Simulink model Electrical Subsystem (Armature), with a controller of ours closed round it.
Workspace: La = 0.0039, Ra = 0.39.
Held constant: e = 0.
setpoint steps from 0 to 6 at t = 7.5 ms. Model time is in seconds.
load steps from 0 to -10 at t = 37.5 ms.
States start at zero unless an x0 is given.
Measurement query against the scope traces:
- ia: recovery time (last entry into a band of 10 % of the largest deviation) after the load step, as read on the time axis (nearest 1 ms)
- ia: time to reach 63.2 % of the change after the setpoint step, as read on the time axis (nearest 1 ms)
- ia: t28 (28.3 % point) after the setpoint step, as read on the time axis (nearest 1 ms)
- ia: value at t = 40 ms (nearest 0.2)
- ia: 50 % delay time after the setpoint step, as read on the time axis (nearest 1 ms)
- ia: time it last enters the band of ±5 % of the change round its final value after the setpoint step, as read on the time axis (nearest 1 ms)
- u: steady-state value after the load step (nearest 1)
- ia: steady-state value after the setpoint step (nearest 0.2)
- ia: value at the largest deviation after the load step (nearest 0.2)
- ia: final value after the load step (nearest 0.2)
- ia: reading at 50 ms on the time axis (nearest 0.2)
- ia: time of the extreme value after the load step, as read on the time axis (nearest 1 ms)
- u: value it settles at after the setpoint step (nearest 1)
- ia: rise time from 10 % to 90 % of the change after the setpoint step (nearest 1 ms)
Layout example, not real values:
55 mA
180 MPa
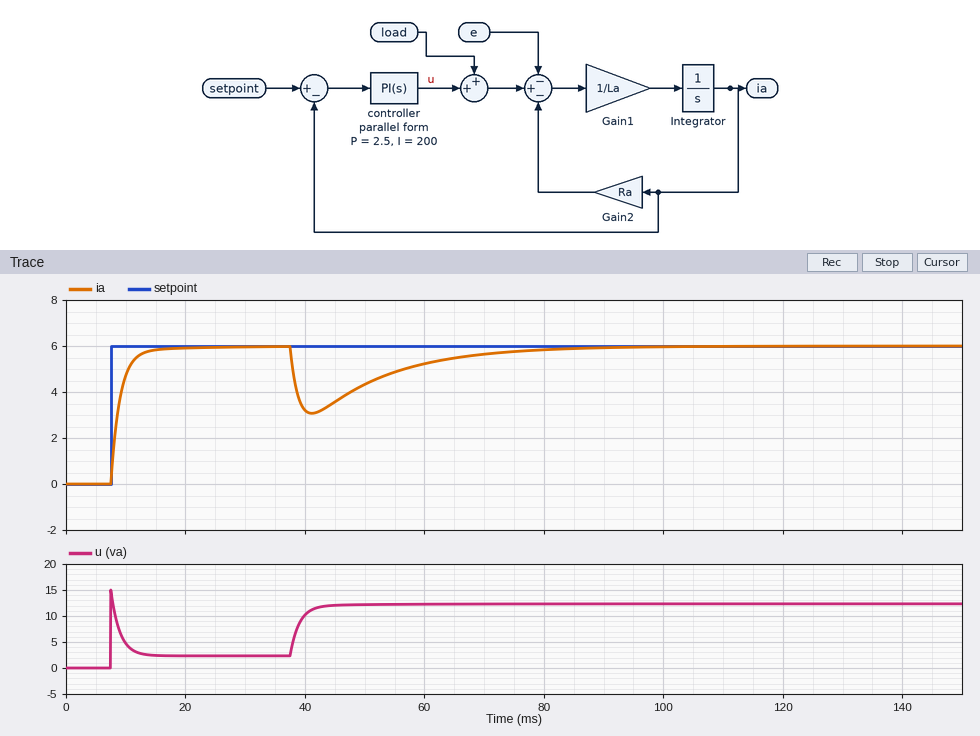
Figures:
73 ms
9 ms
8 ms
3.2
9 ms
13 ms
12
6.0
3.0
6.0
4.4
41 ms
2
4 ms
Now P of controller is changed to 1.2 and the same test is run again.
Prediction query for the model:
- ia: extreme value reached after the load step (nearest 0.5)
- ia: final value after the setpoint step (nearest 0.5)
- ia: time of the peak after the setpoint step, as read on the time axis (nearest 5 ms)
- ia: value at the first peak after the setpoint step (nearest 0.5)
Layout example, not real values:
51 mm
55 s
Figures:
1.5
6.0
20 ms
6.5
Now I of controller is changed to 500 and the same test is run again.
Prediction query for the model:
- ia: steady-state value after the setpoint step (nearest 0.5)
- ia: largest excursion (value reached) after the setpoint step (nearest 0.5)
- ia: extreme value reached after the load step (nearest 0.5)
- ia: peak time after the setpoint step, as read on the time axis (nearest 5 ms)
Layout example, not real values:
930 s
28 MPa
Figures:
6.0
6.5
3.5
15 ms
